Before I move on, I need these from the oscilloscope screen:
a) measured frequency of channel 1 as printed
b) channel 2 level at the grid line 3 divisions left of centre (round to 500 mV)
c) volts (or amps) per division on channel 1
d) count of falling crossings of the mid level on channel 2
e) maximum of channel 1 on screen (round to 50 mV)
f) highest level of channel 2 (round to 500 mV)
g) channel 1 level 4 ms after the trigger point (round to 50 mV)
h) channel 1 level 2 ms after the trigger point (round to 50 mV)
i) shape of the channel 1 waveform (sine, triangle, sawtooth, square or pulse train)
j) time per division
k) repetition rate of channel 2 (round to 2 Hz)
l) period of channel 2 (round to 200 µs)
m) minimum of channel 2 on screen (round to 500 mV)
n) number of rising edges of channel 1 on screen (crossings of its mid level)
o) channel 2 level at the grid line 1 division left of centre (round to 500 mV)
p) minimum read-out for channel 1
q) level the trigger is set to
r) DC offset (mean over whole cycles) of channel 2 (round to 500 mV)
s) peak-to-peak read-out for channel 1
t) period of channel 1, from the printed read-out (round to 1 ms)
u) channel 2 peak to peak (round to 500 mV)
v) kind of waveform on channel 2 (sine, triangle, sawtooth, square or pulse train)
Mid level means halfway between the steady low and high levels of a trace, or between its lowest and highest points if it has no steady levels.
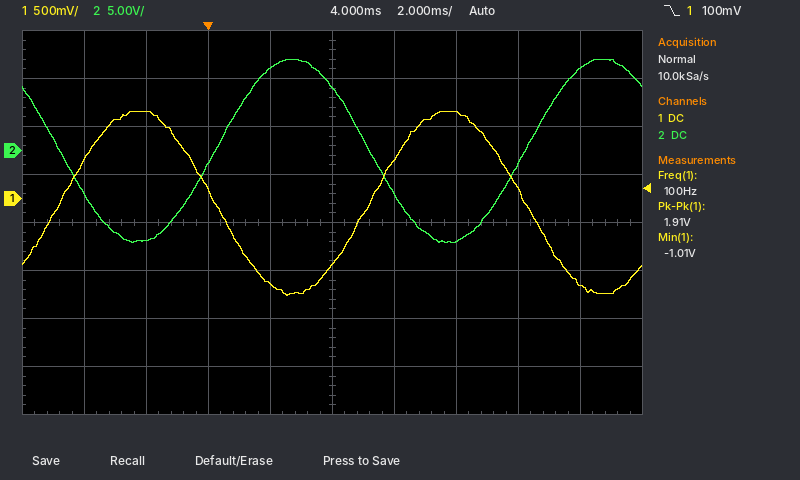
100 Hz
-9.5 V
500 mV
2
900 mV
9.5 V
-700 mV
-900 mV
sine
2 ms
100 Hz
10.0 ms
-9.5 V
2
8.5 V
-1.01 V
100 mV
0.0 V
1.91 V
10 ms
19.0 V
sine
